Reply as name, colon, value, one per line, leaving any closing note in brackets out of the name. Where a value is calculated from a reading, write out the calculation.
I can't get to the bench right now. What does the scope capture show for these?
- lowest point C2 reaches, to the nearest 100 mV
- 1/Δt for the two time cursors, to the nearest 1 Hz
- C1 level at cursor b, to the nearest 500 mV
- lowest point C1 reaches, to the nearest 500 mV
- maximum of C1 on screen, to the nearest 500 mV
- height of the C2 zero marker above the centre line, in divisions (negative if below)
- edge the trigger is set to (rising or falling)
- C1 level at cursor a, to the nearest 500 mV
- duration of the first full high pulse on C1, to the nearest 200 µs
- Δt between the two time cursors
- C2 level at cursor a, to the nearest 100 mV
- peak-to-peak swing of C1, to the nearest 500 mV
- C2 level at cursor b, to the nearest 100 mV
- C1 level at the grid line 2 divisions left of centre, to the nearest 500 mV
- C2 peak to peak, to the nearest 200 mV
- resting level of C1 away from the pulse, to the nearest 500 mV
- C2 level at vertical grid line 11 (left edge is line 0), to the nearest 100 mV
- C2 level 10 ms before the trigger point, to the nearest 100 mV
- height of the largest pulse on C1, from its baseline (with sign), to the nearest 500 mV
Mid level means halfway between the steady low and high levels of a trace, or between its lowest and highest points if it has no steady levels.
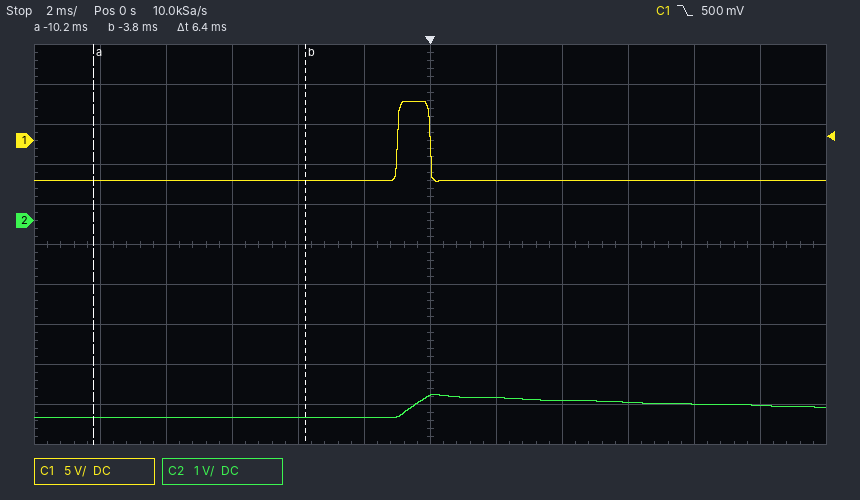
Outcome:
lowest point C2 reaches, to the nearest 100 mV: -4.9 V
1/Δt for the two time cursors, to the nearest 1 Hz: 1 / 6.4 ms ≈ 156 Hz
C1 level at cursor b, to the nearest 500 mV: -5.0 V
lowest point C1 reaches, to the nearest 500 mV: -5.0 V
maximum of C1 on screen, to the nearest 500 mV: 5.0 V
height of the C2 zero marker above the centre line, in divisions: +0.6 div
edge the trigger is set to: falling
C1 level at cursor a, to the nearest 500 mV: -5.0 V
duration of the first full high pulse on C1, to the nearest 200 µs: 1.0 ms
Δt between the two time cursors: 6.4 ms
C2 level at cursor a, to the nearest 100 mV: -4.9 V
peak-to-peak swing of C1, to the nearest 500 mV: 5.0 V − (-5.0 V) = 10.0 V
C2 level at cursor b, to the nearest 100 mV: -4.9 V
C1 level at the grid line 2 divisions left of centre, to the nearest 500 mV: -5.0 V
C2 peak to peak, to the nearest 200 mV: 600 mV
resting level of C1 away from the pulse, to the nearest 500 mV: -5.0 V
C2 level at vertical grid line 11 (left edge is line 0), to the nearest 100 mV: -4.6 V
C2 level 10 ms before the trigger point, to the nearest 100 mV: -4.9 V
height of the largest pulse on C1, from its baseline (with sign), to the nearest 500 mV: 5.0 V − (-5.0 V) = +10.0 V
